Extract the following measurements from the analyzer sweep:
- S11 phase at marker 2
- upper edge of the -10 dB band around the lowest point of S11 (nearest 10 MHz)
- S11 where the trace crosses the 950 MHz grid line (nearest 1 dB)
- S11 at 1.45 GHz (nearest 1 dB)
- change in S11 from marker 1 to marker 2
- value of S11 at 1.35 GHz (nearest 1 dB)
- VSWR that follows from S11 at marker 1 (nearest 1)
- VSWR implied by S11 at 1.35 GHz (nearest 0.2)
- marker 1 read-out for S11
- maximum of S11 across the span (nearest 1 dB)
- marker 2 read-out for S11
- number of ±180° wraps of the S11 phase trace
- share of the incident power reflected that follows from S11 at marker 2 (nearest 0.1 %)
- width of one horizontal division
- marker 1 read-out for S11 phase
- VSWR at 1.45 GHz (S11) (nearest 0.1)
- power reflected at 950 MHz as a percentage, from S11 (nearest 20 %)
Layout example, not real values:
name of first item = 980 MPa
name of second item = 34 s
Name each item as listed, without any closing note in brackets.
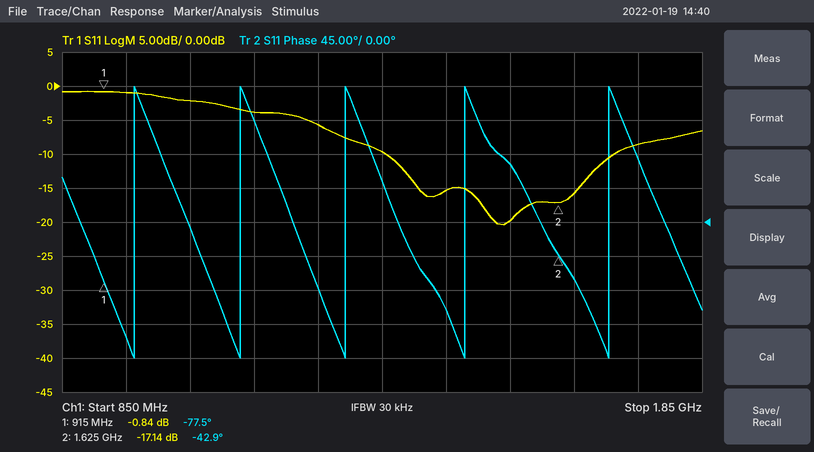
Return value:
S11 phase at marker 2 = -42.9°
upper edge of the -10 dB band around the lowest point of S11 = 1.71 GHz
S11 where the trace crosses the 950 MHz grid line = -1 dB
S11 at 1.45 GHz = -15 dB
change in S11 from marker 1 to marker 2 = -16.30 dB
value of S11 at 1.35 GHz = -10 dB
VSWR that follows from S11 at marker 1 = 21
VSWR implied by S11 at 1.35 GHz = 2.0
marker 1 read-out for S11 = -0.84 dB
maximum of S11 across the span = -1 dB
marker 2 read-out for S11 = -17.14 dB
number of ±180° wraps of the S11 phase trace = 5
share of the incident power reflected that follows from S11 at marker 2 = 1.9 %
width of one horizontal division = 100 MHz
marker 1 read-out for S11 phase = -77.5°
VSWR at 1.45 GHz (S11) = 1.4
power reflected at 950 MHz as a percentage, from S11 = 80 %
